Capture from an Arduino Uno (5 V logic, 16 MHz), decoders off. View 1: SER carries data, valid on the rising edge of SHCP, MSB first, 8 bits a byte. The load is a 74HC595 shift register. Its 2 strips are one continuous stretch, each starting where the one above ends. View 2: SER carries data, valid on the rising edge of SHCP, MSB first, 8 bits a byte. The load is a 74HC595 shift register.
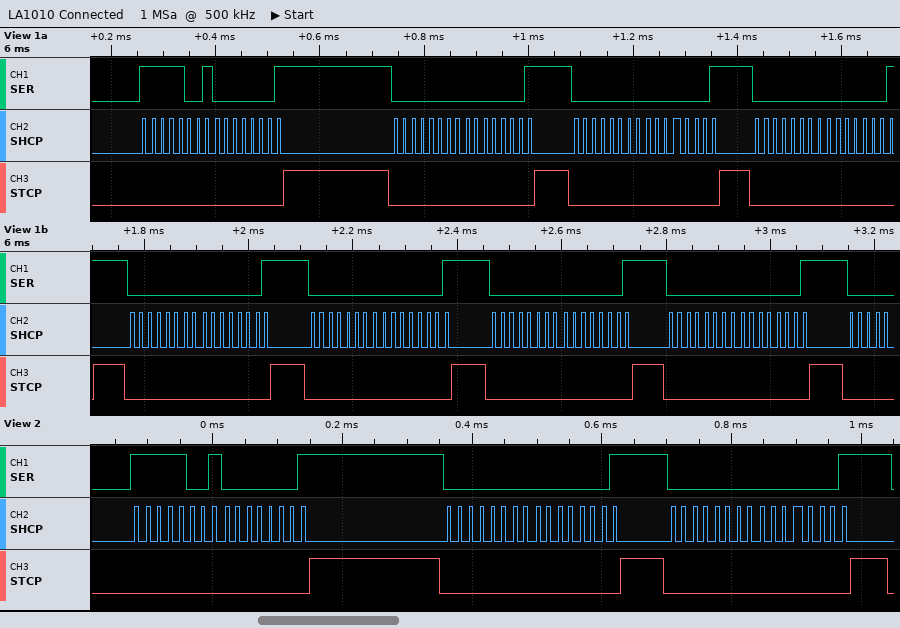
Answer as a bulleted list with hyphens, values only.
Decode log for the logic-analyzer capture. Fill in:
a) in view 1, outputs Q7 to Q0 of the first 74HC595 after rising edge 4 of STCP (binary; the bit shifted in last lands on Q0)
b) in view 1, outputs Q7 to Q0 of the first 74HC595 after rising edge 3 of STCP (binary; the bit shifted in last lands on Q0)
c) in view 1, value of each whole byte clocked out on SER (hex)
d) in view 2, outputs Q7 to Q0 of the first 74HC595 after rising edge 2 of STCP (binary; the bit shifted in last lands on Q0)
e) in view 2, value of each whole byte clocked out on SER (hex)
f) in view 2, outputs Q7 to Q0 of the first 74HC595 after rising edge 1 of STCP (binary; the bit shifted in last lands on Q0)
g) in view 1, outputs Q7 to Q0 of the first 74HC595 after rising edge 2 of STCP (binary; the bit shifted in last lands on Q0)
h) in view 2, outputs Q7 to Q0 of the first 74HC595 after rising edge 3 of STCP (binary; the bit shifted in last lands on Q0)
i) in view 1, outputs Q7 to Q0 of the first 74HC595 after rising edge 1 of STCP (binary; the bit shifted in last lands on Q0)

- 00000001
- 00000001
- F9 01 00 01 00 01 00 01 00 01 00 01 00 01 00 01
- 00000001
- F9 01 00 01 00 01
- 00000001
- 00000001
- 00000001
- 00000001
